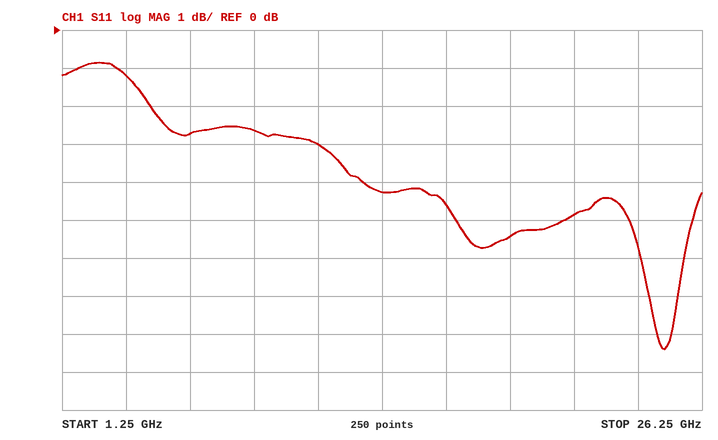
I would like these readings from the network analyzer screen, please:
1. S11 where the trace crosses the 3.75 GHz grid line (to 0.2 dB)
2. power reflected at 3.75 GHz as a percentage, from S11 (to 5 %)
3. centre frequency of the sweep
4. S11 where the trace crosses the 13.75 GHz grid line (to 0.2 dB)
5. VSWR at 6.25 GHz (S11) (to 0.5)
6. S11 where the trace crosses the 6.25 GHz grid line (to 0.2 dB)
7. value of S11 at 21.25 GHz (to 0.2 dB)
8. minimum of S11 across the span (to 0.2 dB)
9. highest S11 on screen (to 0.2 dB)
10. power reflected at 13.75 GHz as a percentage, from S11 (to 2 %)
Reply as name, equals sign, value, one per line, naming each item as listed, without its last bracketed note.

S11 where the trace crosses the 3.75 GHz grid line = -1.2 dB
power reflected at 3.75 GHz as a percentage, from S11 = 75 %
centre frequency of the sweep = 13.75 GHz
S11 where the trace crosses the 13.75 GHz grid line = -4.2 dB
VSWR at 6.25 GHz (S11) = 6.5
S11 where the trace crosses the 6.25 GHz grid line = -2.8 dB
value of S11 at 21.25 GHz = -4.8 dB
minimum of S11 across the span = -8.4 dB
highest S11 on screen = -0.8 dB
power reflected at 13.75 GHz as a percentage, from S11 = 38 %
